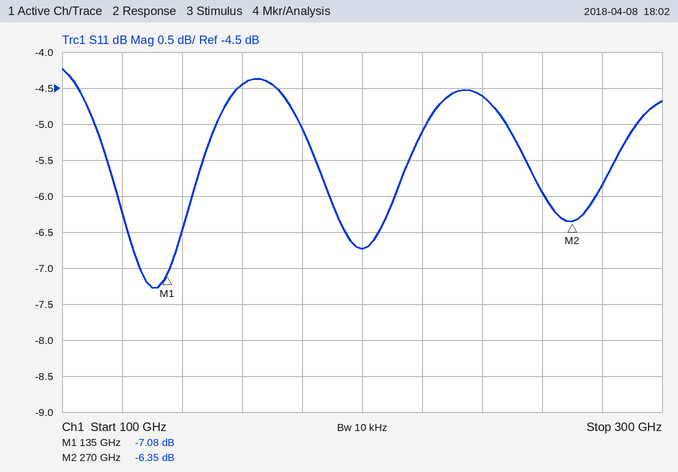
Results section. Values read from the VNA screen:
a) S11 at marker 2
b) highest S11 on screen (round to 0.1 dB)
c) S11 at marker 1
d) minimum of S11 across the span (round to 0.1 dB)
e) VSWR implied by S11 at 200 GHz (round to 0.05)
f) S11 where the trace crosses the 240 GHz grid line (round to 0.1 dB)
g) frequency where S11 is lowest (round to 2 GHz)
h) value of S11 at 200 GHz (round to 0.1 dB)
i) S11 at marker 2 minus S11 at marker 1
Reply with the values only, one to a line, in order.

-6.35 dB
-4.2 dB
-7.08 dB
-7.3 dB
2.70
-4.6 dB
130 GHz
-6.7 dB
0.73 dB
